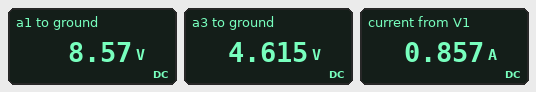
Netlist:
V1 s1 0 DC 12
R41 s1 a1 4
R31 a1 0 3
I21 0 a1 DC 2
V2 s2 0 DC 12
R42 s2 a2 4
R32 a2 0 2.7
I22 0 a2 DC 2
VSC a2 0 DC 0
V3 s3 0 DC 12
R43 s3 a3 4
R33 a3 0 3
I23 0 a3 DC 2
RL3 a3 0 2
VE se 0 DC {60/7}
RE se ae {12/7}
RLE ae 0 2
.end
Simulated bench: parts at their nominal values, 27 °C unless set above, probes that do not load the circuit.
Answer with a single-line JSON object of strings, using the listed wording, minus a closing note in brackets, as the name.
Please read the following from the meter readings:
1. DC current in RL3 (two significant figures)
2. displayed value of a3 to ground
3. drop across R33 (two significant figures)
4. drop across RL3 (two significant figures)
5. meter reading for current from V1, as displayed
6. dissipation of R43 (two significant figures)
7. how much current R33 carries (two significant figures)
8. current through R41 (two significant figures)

{"DC current in RL3": "2.3 A", "displayed value of a3 to ground": "4.615 V", "drop across R33": "4.6 V", "drop across RL3": "4.6 V", "meter reading for current from V1, as displayed": "0.857 A", "dissipation of R43": "14 W", "how much current R33 carries": "1.5 A", "current through R41": "860 mA"}
